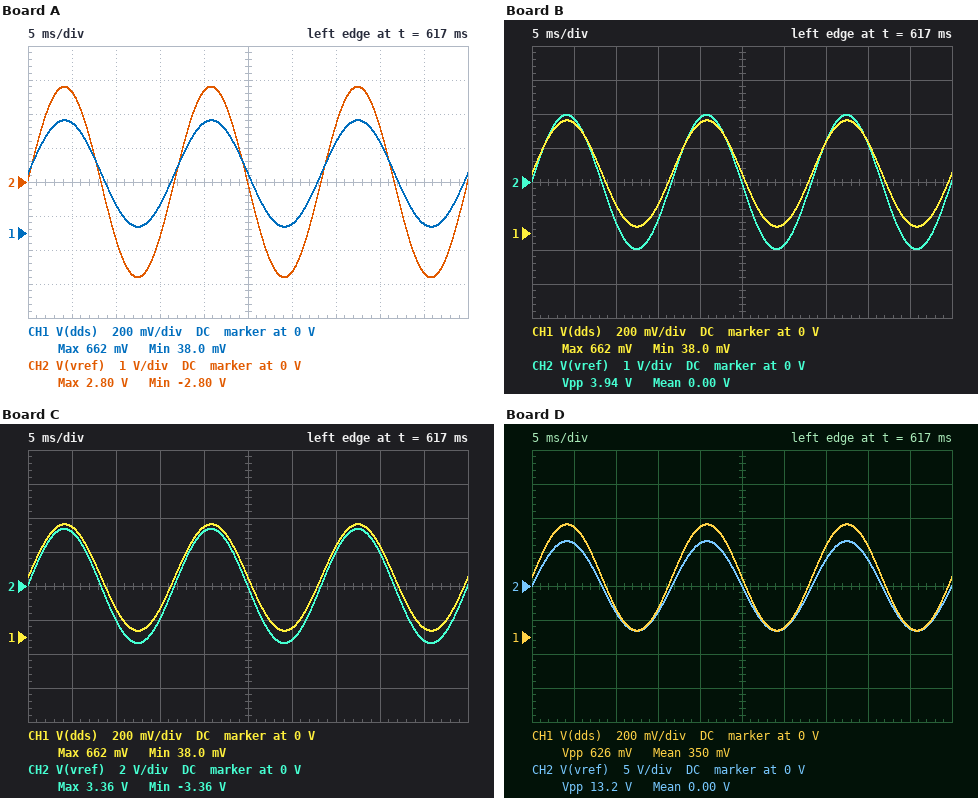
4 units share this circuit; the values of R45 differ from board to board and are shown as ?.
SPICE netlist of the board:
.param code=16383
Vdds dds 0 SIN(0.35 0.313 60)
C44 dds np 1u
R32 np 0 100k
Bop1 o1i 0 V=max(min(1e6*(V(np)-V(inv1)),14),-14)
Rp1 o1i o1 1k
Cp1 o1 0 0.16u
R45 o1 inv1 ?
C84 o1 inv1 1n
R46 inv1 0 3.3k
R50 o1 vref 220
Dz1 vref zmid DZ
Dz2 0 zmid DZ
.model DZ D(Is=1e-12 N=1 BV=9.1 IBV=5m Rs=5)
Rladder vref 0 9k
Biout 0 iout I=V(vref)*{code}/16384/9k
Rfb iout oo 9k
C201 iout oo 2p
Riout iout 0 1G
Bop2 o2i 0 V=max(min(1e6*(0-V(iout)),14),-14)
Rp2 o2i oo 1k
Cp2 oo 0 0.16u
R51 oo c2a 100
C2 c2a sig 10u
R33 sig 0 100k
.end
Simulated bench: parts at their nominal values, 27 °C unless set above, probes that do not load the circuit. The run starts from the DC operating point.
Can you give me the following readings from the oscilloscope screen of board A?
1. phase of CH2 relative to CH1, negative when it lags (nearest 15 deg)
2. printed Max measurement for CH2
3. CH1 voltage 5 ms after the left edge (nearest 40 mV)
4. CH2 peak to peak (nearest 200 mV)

0 deg
2.80 V
640 mV
5.6 V
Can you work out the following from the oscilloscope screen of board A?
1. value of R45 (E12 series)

27 kΩ
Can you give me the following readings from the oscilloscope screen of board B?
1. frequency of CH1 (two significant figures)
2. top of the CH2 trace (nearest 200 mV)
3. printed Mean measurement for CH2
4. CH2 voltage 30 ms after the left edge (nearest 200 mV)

60 Hz
2.0 V
0.00 V
-1.8 V
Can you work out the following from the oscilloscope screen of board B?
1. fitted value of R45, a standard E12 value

18 kΩ
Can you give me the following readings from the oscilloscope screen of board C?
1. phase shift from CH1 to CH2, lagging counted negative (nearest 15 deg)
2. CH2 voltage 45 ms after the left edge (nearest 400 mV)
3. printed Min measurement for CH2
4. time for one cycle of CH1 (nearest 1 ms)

0 deg
-3.2 V
-3.36 V
17 ms
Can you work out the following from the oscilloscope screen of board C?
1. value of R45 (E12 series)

33 kΩ
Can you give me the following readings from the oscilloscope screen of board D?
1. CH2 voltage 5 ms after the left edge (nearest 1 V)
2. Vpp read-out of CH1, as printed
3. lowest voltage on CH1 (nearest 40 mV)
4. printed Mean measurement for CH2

6 V
626 mV
40 mV
0.00 V
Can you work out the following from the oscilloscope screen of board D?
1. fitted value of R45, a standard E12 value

68 kΩ
